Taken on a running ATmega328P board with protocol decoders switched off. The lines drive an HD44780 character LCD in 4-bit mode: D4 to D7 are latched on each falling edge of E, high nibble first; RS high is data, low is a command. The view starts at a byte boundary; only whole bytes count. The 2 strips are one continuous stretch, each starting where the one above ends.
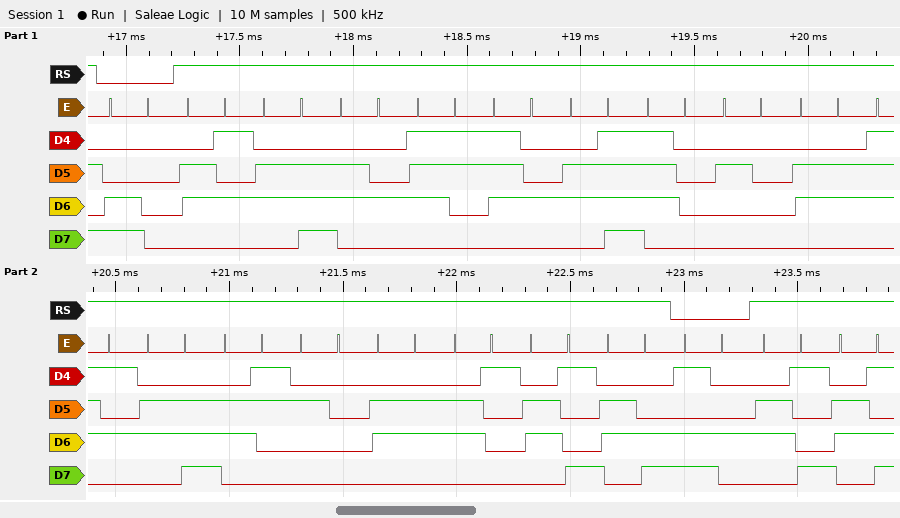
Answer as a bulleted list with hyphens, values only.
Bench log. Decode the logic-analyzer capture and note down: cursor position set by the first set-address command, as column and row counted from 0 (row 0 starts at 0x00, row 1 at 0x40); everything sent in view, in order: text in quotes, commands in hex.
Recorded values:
- column 0, row 1
- 0xC0 "endstop func fail" 0xD4 "im"
